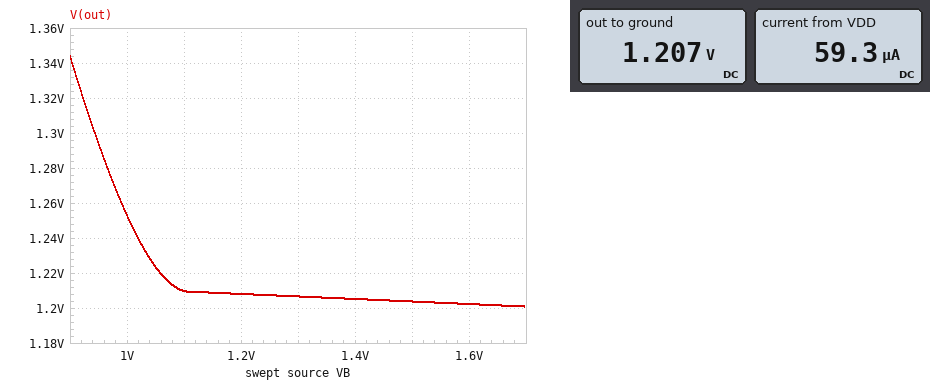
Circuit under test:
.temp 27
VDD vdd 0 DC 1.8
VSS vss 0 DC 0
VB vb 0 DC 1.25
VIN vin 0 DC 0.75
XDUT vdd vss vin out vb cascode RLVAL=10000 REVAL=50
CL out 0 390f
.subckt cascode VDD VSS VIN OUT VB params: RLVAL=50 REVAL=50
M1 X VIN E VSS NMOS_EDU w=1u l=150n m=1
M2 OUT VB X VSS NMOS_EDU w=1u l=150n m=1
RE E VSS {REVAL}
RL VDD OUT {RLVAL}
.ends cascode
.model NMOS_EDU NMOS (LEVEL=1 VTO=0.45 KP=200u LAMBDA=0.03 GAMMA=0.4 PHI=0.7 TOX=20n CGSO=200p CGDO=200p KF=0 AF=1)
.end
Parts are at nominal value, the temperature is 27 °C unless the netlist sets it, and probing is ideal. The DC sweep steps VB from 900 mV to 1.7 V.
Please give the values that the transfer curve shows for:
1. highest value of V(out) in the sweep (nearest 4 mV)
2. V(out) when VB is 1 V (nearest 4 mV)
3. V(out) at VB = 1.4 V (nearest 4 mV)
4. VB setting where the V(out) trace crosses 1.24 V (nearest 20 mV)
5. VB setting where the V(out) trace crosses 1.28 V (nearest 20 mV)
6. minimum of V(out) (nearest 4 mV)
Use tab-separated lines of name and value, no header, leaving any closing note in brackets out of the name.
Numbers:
highest value of V(out) in the sweep	1.344 V
V(out) when VB is 1 V	1.252 V
V(out) at VB = 1.4 V	1.204 V
VB setting where the V(out) trace crosses 1.24 V	1.02 V
VB setting where the V(out) trace crosses 1.28 V	960 mV
minimum of V(out)	1.200 V
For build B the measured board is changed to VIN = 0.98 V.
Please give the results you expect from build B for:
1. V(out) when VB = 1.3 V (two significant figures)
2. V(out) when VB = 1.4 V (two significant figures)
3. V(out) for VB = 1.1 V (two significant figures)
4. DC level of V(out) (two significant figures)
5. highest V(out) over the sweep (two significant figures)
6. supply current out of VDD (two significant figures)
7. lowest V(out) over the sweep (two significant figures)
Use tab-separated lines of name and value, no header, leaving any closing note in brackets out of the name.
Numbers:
V(out) when VB = 1.3 V	480 mV
V(out) when VB = 1.4 V	450 mV
V(out) for VB = 1.1 V	690 mV
DC level of V(out)	510 mV
highest V(out) over the sweep	1.1 V
supply current out of VDD	130 µA
lowest V(out) over the sweep	400 mV
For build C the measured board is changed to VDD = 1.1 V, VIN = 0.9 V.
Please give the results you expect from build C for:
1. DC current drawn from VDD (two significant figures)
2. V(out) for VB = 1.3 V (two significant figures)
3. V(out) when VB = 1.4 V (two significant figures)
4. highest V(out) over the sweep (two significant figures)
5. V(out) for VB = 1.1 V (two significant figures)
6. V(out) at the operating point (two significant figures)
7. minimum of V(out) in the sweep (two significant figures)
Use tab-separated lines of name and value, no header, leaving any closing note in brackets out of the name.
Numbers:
DC current drawn from VDD	81 µA
V(out) for VB = 1.3 V	280 mV
V(out) when VB = 1.4 V	270 mV
highest V(out) over the sweep	490 mV
V(out) for VB = 1.1 V	320 mV
V(out) at the operating point	290 mV
minimum of V(out) in the sweep	250 mV
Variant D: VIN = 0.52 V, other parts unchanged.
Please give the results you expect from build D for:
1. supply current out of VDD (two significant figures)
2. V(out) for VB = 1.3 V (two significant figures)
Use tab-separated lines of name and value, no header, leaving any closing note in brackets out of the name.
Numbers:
supply current out of VDD	3.3 µA
V(out) for VB = 1.3 V	1.8 V
